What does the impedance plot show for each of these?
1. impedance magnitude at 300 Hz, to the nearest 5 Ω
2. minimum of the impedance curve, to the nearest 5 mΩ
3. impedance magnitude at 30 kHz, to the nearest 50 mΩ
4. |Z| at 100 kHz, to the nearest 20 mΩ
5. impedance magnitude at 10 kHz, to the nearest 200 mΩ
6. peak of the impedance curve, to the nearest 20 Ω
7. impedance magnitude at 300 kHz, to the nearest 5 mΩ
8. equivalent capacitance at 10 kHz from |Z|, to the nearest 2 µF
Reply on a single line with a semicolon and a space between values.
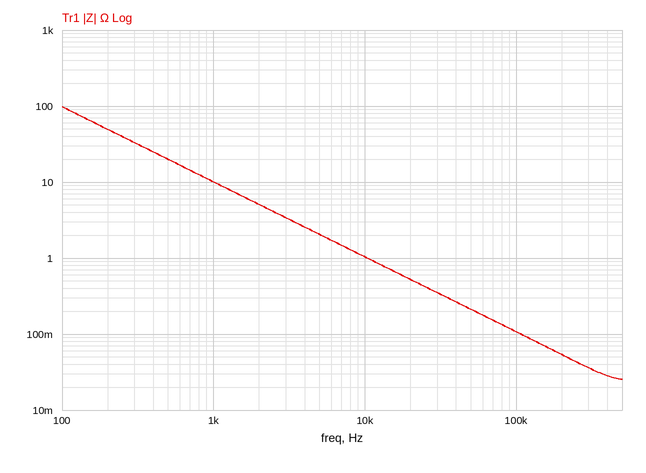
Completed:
35 Ω; 25 mΩ; 350 mΩ; 100 mΩ; 1.0 Ω; 100 Ω; 35 mΩ; 16 µF
